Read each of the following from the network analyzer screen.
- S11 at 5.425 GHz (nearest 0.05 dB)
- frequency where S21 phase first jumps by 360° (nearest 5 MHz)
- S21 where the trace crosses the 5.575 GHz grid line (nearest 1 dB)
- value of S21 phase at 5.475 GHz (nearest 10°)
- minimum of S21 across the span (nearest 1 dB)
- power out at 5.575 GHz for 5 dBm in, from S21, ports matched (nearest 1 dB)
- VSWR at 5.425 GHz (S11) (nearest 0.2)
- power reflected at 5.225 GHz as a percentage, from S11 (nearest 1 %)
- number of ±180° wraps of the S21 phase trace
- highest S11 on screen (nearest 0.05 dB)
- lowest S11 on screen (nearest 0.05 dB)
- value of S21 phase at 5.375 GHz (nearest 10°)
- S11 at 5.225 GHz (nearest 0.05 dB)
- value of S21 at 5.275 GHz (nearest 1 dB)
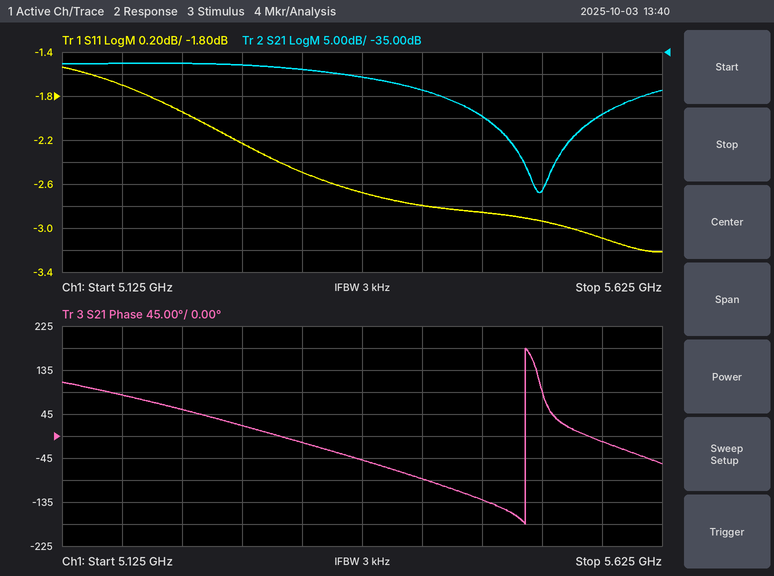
-2.80 dB
5.510 GHz
-49 dB
-130°
-67 dB
-44 dBm
6.2
64 %
1
-1.55 dB
-3.20 dB
-50°
-1.95 dB
-38 dB
